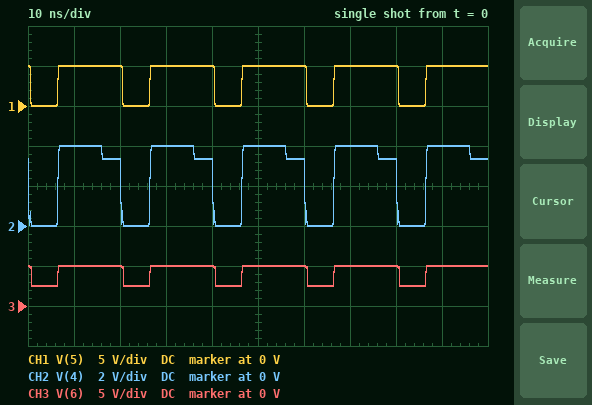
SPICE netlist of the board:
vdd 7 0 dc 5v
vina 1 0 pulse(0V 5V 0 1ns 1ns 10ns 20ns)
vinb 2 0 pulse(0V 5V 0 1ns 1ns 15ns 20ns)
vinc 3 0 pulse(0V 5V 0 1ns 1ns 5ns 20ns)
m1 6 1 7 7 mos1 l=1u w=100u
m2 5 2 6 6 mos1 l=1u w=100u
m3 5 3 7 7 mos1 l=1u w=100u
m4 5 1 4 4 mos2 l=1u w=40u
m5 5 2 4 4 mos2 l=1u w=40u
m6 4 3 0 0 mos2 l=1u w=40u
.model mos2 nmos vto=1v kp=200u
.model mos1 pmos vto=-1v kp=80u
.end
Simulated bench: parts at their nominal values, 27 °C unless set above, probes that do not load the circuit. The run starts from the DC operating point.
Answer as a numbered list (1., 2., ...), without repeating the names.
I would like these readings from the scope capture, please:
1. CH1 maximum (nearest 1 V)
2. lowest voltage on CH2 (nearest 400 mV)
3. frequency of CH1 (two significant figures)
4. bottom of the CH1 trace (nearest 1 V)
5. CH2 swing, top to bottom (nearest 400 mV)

1. 5 V
2. 0 V
3. 50 MHz
4. 0 V
5. 4.0 V
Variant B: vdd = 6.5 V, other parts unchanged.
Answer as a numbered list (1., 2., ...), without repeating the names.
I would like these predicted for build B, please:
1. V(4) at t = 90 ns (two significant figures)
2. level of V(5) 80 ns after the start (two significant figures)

1. 4.3 V
2. 6.5 V
